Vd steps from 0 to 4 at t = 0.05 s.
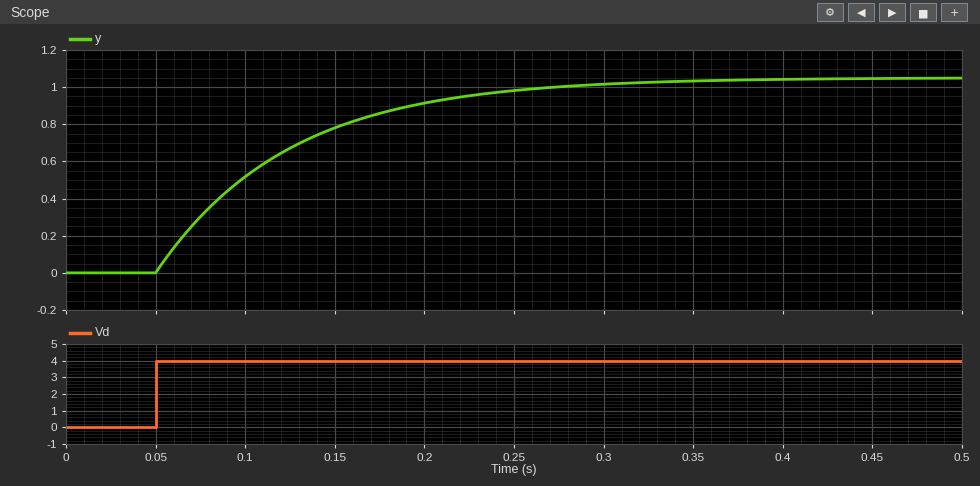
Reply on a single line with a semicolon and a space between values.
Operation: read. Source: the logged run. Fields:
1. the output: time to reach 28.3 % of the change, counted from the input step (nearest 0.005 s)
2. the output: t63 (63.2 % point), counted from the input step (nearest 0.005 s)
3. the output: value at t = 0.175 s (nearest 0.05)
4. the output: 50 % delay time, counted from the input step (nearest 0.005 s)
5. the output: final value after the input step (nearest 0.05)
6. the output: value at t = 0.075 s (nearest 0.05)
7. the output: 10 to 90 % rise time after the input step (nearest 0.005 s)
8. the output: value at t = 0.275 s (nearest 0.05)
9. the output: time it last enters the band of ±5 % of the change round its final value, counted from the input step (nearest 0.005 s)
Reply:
0.025 s; 0.075 s; 0.85; 0.050 s; 1.05; 0.30; 0.160 s; 1.00; 0.220 s
